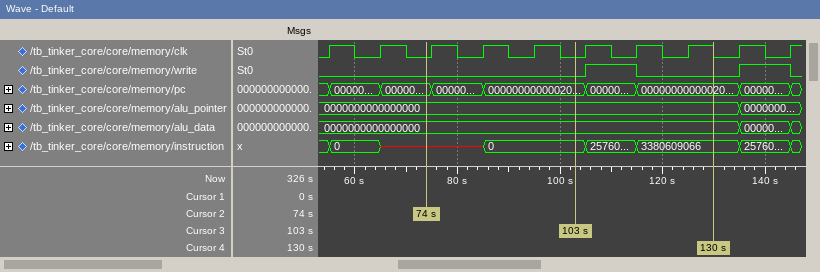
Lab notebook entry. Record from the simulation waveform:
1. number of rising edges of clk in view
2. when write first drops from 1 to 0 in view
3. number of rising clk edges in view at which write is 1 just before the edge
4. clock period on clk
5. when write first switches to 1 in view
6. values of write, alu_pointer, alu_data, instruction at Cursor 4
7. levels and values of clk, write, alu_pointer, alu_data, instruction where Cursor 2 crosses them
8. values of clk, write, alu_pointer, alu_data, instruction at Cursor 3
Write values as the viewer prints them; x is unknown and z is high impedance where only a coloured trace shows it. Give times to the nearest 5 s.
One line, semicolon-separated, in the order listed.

10; 115 s; 2; 10 s; 105 s; write=0, alu_pointer=0000000000000000, alu_data=0000000000000000, instruction=3380609066; clk=0, write=0, alu_pointer=0000000000000000, alu_data=0000000000000000, instruction=x; clk=0, write=0, alu_pointer=0000000000000000, alu_data=0000000000000000, instruction=0
